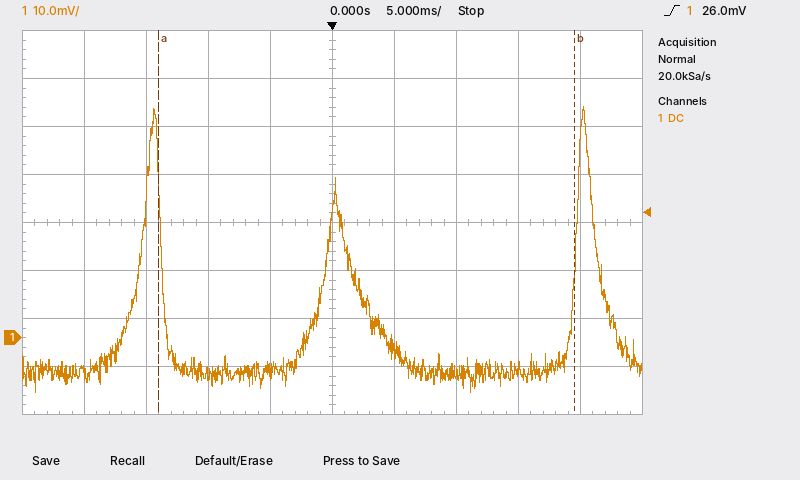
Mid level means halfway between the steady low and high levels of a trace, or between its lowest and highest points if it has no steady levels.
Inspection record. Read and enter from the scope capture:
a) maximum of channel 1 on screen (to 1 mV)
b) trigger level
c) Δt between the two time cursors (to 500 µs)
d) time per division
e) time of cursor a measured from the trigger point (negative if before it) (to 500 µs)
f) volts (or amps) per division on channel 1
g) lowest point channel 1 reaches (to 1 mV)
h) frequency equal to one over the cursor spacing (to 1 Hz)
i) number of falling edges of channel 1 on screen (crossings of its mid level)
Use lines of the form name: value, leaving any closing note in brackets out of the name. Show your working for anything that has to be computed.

maximum of channel 1 on screen: 48 mV
trigger level: 26.0 mV
Δt between the two time cursors: 33.5 ms
time per division: 5 ms
time of cursor a measured from the trigger point (negative if before it): -14.0 ms
volts (or amps) per division on channel 1: 10 mV
lowest point channel 1 reaches: -11 mV
frequency equal to one over the cursor spacing: 1 / 33.5 ms ≈ 30 Hz
number of falling edges of channel 1 on screen: 3
